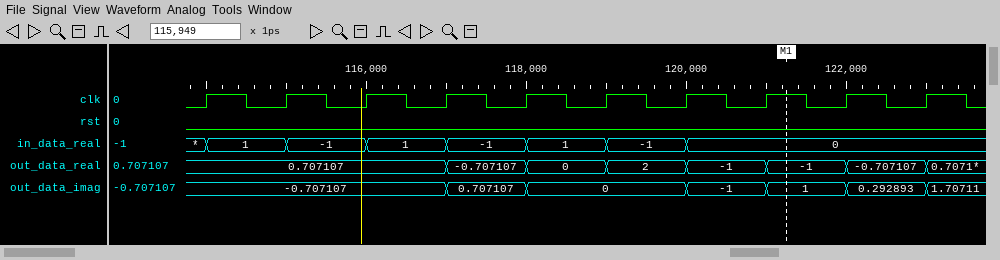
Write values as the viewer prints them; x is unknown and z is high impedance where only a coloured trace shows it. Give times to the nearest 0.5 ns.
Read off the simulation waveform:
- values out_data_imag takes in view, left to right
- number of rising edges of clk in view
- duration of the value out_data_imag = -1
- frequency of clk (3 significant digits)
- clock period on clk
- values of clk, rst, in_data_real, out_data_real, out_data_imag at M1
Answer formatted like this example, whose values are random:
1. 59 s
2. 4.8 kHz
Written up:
1. -0.707107, 0.707107, 0, -1, 1, 0.292893, 1.70711
2. 10
3. 1 ns
4. 1.00 GHz
5. 1 ns
6. clk=1, rst=0, in_data_real=0, out_data_real=-1, out_data_imag=1
